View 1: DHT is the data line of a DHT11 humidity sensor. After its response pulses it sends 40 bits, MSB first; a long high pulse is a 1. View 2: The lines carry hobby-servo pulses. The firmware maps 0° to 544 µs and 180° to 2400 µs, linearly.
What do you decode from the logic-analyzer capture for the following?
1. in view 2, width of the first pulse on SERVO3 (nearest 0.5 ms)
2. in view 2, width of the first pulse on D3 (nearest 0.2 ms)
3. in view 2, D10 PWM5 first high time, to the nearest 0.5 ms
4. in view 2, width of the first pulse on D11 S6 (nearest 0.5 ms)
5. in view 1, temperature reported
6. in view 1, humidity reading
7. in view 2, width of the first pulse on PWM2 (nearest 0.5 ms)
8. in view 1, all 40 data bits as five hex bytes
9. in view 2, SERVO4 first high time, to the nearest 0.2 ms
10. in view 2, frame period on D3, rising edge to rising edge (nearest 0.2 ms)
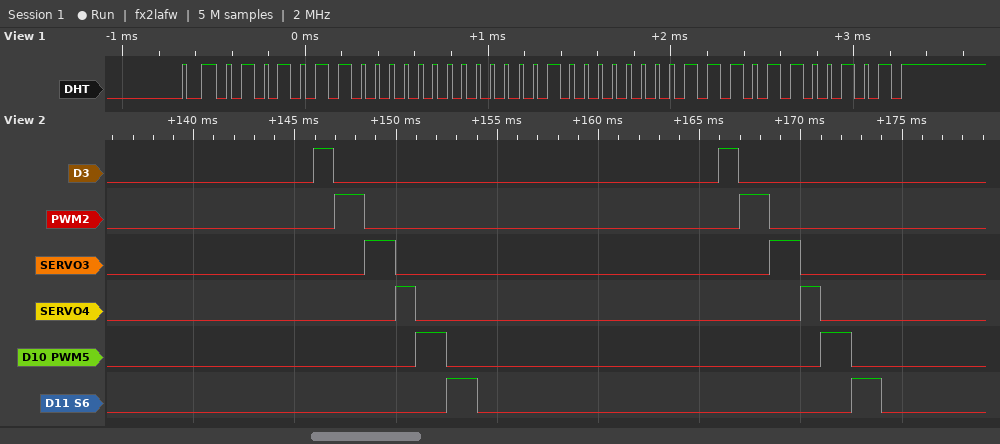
1.5 ms
1.0 ms
1.5 ms
1.5 ms
8.7 °C
86 %
1.5 ms
56 00 08 07 65
1.0 ms
20.0 ms
